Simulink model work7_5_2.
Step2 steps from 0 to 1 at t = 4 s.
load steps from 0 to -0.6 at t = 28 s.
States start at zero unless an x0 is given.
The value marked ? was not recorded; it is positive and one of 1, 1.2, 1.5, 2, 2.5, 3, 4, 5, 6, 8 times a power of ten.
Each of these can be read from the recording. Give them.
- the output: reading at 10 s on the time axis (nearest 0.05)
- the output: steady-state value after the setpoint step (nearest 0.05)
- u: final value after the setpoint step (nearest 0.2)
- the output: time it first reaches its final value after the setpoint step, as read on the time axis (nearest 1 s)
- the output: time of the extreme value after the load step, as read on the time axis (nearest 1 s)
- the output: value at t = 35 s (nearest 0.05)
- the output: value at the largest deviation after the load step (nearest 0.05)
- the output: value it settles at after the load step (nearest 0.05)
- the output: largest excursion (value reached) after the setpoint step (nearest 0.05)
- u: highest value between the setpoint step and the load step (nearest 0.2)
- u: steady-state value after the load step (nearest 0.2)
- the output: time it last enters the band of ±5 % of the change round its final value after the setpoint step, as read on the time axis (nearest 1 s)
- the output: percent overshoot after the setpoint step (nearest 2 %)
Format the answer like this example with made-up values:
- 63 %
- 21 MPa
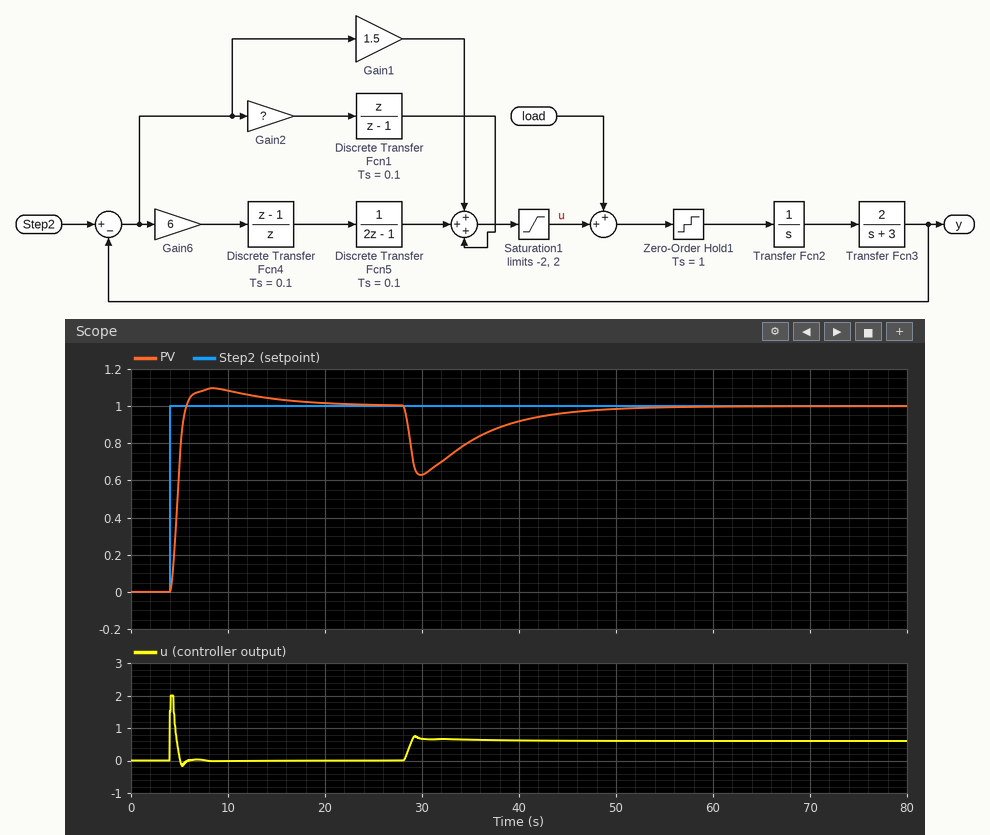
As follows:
- 1.10
- 1.00
- 0.0
- 6 s
- 30 s
- 0.80
- 0.65
- 1.00
- 1.10
- 2.0
- 0.6
- 13 s
- 10 %
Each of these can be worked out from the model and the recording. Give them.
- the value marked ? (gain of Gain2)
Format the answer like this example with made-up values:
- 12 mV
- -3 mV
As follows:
- 0.02
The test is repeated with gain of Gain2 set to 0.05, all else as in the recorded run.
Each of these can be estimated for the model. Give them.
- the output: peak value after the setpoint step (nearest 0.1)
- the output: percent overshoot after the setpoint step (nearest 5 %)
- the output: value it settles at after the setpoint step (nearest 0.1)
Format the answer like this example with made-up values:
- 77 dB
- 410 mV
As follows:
- 1.2
- 20 %
- 1.0
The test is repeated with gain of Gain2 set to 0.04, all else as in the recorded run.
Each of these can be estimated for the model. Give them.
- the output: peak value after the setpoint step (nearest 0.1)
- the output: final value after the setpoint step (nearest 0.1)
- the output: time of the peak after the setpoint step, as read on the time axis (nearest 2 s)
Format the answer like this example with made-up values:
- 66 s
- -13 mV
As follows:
- 1.2
- 1.0
- 8 s
